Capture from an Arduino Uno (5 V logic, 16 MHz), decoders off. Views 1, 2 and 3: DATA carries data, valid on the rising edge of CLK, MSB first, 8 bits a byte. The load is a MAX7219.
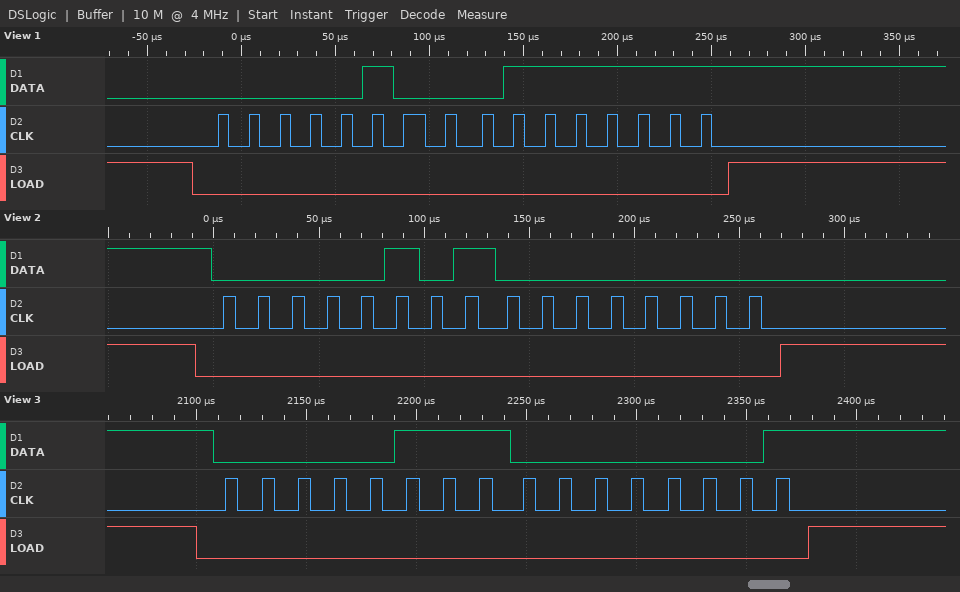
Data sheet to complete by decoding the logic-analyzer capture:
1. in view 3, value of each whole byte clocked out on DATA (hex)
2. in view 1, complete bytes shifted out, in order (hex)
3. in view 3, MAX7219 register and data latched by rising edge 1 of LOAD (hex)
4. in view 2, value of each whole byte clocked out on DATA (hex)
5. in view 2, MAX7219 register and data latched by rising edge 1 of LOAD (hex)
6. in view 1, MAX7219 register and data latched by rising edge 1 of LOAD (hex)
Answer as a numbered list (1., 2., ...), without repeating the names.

1. 0x07 0x01
2. 04 7F
3. register 0x7, data 0x01
4. 05 00
5. register 0x5, data 0x00
6. register 0x4, data 0x7F
